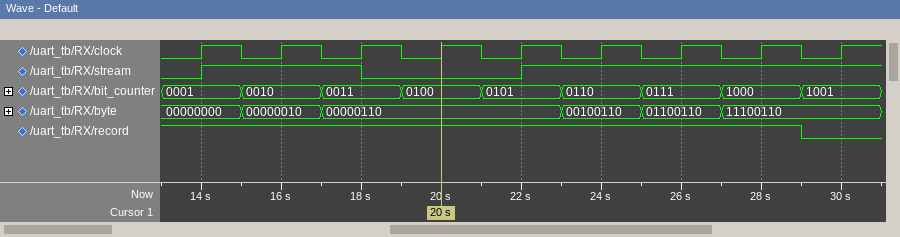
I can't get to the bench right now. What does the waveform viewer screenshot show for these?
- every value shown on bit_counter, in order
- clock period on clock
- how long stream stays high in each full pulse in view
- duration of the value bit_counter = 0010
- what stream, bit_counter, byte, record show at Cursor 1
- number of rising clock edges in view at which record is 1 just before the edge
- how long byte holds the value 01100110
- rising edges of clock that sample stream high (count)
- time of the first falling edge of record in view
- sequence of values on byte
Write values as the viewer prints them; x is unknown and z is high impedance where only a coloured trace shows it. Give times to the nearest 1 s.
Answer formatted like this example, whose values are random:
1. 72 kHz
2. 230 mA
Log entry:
1. 0001, 0010, 0011, 0100, 0101, 0110, 0111, 1000, 1001
2. 2 s
3. 4 s
4. 2 s
5. stream=0, bit_counter=0100, byte=00000110, record=1
6. 8
7. 2 s
8. 6
9. 29 s
10. 00000000, 00000010, 00000110, 00100110, 01100110, 11100110
